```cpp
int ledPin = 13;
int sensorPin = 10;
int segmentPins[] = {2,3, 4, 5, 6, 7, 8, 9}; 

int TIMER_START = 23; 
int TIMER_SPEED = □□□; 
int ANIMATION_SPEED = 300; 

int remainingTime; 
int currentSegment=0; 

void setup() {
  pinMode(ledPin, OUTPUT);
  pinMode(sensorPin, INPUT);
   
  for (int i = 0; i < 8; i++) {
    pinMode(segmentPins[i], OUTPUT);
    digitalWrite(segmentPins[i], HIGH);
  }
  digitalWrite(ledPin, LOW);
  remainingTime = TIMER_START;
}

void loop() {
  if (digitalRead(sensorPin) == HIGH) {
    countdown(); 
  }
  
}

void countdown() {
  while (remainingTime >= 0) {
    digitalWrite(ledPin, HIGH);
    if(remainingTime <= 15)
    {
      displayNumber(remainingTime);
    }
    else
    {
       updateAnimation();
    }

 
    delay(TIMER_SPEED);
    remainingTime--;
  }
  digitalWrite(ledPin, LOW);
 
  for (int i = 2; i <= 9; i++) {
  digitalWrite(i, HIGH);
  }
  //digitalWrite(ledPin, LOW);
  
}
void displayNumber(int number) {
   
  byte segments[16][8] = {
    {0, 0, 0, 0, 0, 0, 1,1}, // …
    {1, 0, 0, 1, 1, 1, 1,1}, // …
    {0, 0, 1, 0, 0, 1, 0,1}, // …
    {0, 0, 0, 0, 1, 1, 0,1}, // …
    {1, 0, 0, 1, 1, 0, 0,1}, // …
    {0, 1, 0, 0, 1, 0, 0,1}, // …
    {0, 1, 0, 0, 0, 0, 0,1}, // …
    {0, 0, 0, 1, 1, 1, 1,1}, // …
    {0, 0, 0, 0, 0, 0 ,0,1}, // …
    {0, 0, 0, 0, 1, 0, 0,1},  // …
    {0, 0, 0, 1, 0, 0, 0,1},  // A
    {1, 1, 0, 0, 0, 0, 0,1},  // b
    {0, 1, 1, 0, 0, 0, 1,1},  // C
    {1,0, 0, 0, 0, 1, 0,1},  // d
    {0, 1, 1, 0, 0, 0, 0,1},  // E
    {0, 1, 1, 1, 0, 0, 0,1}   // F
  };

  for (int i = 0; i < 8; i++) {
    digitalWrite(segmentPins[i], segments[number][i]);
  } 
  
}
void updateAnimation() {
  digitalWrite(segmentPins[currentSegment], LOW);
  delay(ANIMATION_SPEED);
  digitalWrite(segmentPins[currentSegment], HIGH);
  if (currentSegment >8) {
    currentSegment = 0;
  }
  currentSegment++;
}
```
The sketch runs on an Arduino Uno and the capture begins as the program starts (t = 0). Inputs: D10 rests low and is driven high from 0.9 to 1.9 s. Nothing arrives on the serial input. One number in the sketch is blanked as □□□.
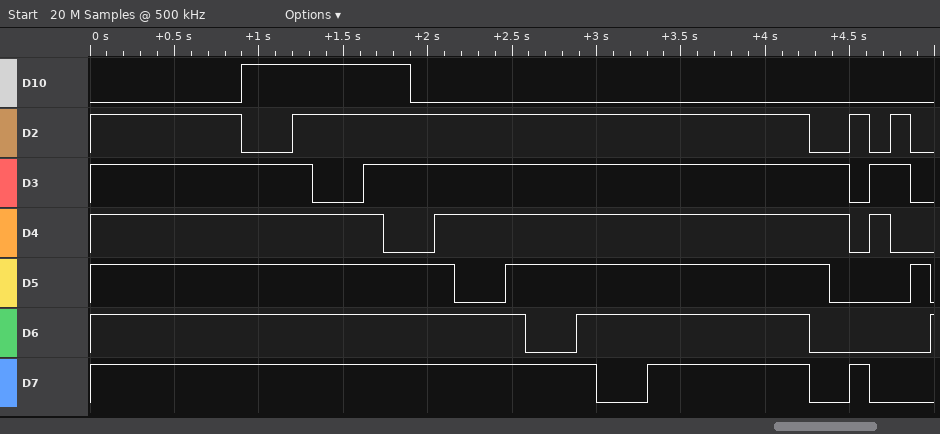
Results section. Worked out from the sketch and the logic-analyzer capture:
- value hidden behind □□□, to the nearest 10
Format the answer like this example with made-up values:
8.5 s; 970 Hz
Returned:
120
